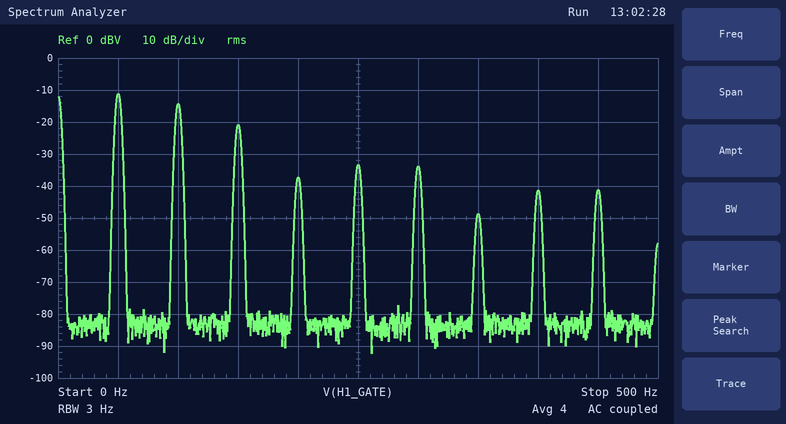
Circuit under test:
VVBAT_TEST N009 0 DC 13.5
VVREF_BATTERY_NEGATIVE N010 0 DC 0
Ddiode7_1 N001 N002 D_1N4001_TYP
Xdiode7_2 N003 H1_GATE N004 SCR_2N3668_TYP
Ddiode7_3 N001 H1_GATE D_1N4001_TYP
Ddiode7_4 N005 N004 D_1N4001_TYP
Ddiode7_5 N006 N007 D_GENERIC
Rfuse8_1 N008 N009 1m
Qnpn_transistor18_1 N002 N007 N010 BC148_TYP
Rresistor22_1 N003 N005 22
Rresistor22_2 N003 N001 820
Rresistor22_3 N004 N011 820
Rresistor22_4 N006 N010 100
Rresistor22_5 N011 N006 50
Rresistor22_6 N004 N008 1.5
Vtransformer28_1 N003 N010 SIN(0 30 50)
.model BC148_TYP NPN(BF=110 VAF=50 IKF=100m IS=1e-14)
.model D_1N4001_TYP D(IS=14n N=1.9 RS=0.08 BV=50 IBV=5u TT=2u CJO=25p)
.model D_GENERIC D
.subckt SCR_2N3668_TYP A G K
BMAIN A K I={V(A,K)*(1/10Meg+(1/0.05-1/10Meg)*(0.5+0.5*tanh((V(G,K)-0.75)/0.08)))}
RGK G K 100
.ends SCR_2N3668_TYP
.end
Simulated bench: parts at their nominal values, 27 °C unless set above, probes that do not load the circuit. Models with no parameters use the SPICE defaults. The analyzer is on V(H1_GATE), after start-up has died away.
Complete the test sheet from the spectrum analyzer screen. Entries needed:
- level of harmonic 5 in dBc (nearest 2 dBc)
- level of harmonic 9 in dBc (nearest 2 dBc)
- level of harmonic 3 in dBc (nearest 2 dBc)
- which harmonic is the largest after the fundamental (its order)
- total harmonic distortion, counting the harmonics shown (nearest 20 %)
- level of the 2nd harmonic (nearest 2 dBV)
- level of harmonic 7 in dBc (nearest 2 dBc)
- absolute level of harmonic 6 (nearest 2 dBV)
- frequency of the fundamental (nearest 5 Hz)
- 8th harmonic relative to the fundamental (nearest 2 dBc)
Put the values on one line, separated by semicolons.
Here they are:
-22 dBc; -30 dBc; -10 dBc; 2; 80 %; -14 dBV; -38 dBc; -34 dBV; 50 Hz; -30 dBc
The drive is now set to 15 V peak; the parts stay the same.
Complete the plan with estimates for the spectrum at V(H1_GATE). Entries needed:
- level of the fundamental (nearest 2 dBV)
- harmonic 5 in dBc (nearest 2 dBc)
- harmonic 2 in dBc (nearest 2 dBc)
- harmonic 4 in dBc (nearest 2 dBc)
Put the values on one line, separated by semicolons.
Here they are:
-46 dBV; -2 dBc; 0 dBc; -2 dBc
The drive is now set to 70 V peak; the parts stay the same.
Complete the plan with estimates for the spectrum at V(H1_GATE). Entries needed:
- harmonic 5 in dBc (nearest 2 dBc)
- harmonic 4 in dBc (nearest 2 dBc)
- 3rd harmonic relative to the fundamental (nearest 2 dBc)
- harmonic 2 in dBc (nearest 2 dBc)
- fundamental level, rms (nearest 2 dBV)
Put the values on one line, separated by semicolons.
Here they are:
-24 dBc; -20 dBc; -12 dBc; -16 dBc; 8 dBV
